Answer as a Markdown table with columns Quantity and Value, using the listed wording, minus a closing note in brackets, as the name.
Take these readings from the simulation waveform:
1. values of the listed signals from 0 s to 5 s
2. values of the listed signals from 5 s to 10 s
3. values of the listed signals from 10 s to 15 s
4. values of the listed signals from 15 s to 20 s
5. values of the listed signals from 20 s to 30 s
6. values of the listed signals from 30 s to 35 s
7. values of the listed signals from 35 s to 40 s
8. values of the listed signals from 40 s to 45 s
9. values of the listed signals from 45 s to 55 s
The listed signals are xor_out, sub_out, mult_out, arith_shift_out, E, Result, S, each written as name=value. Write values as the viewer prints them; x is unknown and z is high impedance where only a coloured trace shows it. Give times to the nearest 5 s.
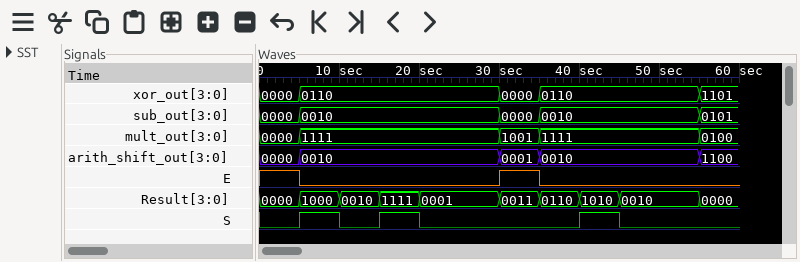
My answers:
| Quantity | Value |
|---|---|
| values of the listed signals from 0 s to 5 s | xor_out=0000, sub_out=0000, mult_out=0000, arith_shift_out=0000, E=1, Result=0000, S=0 |
| values of the listed signals from 5 s to 10 s | xor_out=0110, sub_out=0010, mult_out=1111, arith_shift_out=0010, E=0, Result=1000, S=1 |
| values of the listed signals from 10 s to 15 s | xor_out=0110, sub_out=0010, mult_out=1111, arith_shift_out=0010, E=0, Result=0010, S=0 |
| values of the listed signals from 15 s to 20 s | xor_out=0110, sub_out=0010, mult_out=1111, arith_shift_out=0010, E=0, Result=1111, S=1 |
| values of the listed signals from 20 s to 30 s | xor_out=0110, sub_out=0010, mult_out=1111, arith_shift_out=0010, E=0, Result=0001, S=0 |
| values of the listed signals from 30 s to 35 s | xor_out=0000, sub_out=0000, mult_out=1001, arith_shift_out=0001, E=1, Result=0011, S=0 |
| values of the listed signals from 35 s to 40 s | xor_out=0110, sub_out=0010, mult_out=1111, arith_shift_out=0010, E=0, Result=0110, S=0 |
| values of the listed signals from 40 s to 45 s | xor_out=0110, sub_out=0010, mult_out=1111, arith_shift_out=0010, E=0, Result=1010, S=1 |
| values of the listed signals from 45 s to 55 s | xor_out=0110, sub_out=0010, mult_out=1111, arith_shift_out=0010, E=0, Result=0010, S=0 |
